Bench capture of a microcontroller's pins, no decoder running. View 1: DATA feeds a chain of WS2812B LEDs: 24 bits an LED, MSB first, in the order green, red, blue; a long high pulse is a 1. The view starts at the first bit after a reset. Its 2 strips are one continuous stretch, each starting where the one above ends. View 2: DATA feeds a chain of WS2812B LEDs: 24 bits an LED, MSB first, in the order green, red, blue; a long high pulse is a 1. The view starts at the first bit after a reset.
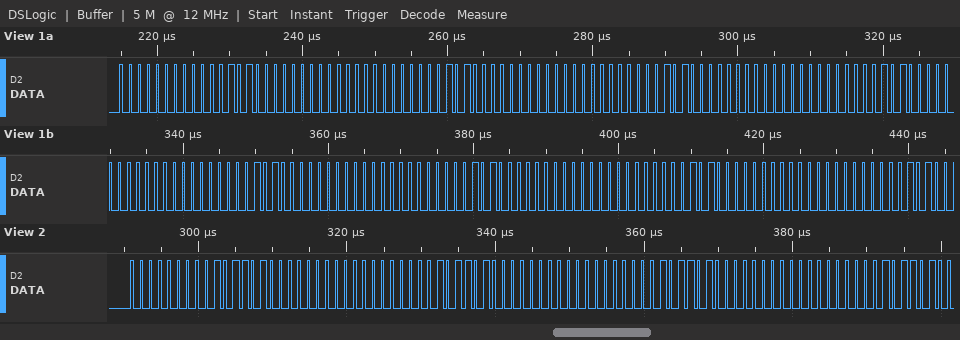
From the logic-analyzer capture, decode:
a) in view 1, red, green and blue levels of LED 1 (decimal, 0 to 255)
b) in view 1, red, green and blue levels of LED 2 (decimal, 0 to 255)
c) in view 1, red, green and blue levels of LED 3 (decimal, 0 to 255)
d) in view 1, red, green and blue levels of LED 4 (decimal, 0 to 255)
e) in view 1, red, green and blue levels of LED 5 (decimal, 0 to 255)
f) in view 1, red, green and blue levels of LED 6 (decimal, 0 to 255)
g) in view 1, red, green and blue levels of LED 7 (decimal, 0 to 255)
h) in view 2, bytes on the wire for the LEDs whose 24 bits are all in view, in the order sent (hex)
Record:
10, 0, 0
10, 0, 0
10, 0, 0
10, 0, 0
10, 0, 0
10, 0, 0
10, 0, 0
00 5A 00 00 5A 00 00 5A 00
